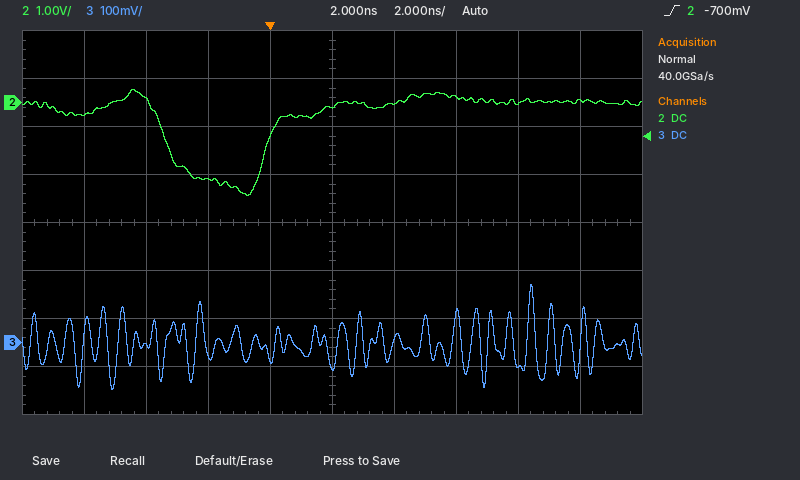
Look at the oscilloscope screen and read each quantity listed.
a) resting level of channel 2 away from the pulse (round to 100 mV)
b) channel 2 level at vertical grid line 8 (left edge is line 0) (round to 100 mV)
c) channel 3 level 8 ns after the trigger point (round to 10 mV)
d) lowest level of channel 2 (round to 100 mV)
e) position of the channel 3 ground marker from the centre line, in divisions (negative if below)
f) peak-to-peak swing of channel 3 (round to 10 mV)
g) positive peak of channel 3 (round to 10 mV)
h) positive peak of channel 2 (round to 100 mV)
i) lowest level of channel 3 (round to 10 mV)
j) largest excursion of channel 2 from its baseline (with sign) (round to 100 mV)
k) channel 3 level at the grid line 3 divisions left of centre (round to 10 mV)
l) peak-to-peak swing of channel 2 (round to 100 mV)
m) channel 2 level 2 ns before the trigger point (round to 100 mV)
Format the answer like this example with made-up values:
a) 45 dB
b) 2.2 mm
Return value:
a) 0.0 V
b) 0.0 V
c) -40 mV
d) -1.9 V
e) -2.5 div
f) 220 mV
g) 120 mV
h) 300 mV
i) -100 mV
j) -1.9 V
k) -10 mV
l) 2.2 V
m) -1.6 V
